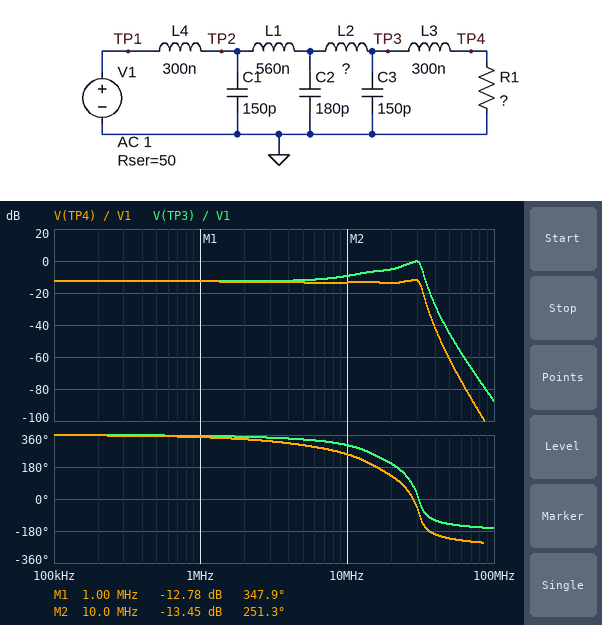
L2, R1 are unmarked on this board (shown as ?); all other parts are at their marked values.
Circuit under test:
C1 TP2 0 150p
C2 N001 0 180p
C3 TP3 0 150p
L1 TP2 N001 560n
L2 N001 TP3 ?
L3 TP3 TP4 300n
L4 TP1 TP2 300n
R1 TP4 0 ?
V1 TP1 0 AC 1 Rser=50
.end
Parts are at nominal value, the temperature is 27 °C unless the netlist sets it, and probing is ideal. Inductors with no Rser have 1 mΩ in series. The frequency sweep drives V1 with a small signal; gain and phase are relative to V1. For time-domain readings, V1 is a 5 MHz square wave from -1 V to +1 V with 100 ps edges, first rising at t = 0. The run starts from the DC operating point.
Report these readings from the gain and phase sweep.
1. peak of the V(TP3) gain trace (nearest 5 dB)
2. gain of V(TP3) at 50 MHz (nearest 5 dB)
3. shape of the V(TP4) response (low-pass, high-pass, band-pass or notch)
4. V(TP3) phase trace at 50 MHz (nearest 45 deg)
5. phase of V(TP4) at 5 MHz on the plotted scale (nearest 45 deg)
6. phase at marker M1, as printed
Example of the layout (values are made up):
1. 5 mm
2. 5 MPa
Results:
1. 0 dB
2. -45 dB
3. low-pass
4. -135 deg
5. 315 deg
6. 347.9 deg
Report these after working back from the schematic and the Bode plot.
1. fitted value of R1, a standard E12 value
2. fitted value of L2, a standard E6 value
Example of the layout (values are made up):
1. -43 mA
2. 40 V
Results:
1. 15 Ω
2. 680 nH
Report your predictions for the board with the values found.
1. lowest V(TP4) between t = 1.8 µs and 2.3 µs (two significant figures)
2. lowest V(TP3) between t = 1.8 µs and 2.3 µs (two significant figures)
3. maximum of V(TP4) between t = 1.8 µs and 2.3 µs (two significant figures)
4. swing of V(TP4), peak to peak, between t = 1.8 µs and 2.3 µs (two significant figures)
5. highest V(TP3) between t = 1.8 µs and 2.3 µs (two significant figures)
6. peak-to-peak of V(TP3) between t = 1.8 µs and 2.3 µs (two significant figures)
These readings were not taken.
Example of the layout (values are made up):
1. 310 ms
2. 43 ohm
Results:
1. -280 mV
2. -610 mV
3. 280 mV
4. 550 mV
5. 610 mV
6. 1.2 V
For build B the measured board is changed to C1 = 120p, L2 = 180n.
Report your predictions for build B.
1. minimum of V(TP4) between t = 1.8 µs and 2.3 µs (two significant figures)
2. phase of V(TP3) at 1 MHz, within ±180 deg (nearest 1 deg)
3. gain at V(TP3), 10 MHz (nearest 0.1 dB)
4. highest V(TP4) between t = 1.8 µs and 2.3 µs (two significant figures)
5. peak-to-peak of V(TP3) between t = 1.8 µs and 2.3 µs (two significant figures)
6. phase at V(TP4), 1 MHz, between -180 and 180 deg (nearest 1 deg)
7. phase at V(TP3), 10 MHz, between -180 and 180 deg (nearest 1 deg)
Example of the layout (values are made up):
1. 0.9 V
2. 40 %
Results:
1. -290 mV
2. -2 deg
3. -8.6 dB
4. 290 mV
5. 1.4 V
6. -9 deg
7. -34 deg
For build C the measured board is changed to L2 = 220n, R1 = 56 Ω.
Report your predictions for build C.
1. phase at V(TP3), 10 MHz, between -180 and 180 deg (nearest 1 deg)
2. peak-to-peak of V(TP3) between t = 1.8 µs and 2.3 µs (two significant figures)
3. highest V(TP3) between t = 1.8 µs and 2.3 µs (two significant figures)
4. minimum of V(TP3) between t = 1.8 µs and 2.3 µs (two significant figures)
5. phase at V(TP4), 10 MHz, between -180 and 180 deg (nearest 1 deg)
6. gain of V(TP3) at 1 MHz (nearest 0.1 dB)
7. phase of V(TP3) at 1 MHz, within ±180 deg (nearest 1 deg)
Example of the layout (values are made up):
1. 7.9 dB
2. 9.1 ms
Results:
1. -77 deg
2. 1.4 V
3. 720 mV
4. -720 mV
5. -95 deg
6. -5.5 dB
7. -7 deg
